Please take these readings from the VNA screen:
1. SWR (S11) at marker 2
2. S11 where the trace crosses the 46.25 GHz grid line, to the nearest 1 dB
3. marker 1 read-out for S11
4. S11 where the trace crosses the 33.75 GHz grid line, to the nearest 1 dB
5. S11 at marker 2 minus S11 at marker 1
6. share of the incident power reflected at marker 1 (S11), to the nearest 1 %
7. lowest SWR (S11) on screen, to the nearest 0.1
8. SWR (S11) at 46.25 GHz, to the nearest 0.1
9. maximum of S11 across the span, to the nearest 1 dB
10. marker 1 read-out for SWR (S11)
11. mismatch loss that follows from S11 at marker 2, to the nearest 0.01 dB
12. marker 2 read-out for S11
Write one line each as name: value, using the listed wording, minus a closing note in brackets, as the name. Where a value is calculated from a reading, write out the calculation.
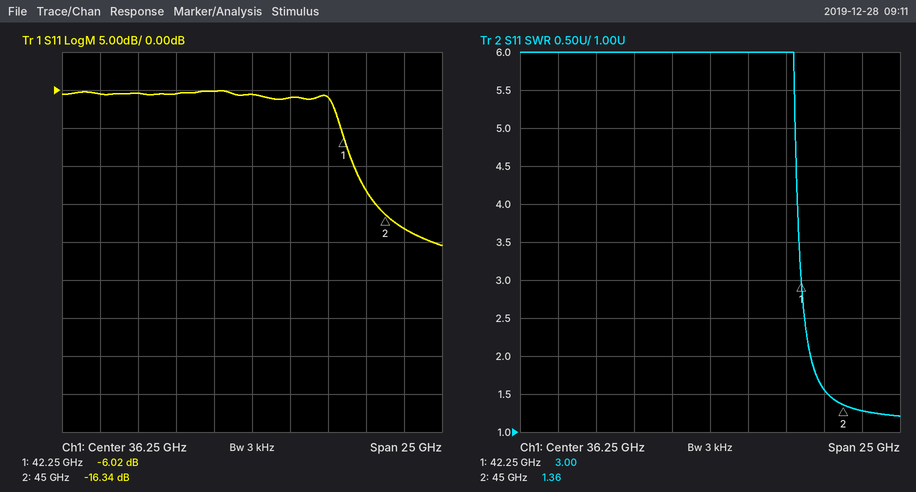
SWR (S11) at marker 2: 1.36
S11 where the trace crosses the 46.25 GHz grid line, to the nearest 1 dB: -18 dB
marker 1 read-out for S11: -6.02 dB
S11 where the trace crosses the 33.75 GHz grid line, to the nearest 1 dB: 0 dB
S11 at marker 2 minus S11 at marker 1: -16.34 − (-6.02) = -10.32 dB
share of the incident power reflected at marker 1 (S11), to the nearest 1 %: 10^(-6.02/10) ≈ 25 %
lowest SWR (S11) on screen, to the nearest 0.1: 1.2
SWR (S11) at 46.25 GHz, to the nearest 0.1: 1.3
maximum of S11 across the span, to the nearest 1 dB: 0 dB
marker 1 read-out for SWR: 3.00
mismatch loss that follows from S11 at marker 2, to the nearest 0.01 dB: −10 log10(1 − 10^(-16.34/10)) ≈ 0.10 dB
marker 2 read-out for S11: -16.34 dB
